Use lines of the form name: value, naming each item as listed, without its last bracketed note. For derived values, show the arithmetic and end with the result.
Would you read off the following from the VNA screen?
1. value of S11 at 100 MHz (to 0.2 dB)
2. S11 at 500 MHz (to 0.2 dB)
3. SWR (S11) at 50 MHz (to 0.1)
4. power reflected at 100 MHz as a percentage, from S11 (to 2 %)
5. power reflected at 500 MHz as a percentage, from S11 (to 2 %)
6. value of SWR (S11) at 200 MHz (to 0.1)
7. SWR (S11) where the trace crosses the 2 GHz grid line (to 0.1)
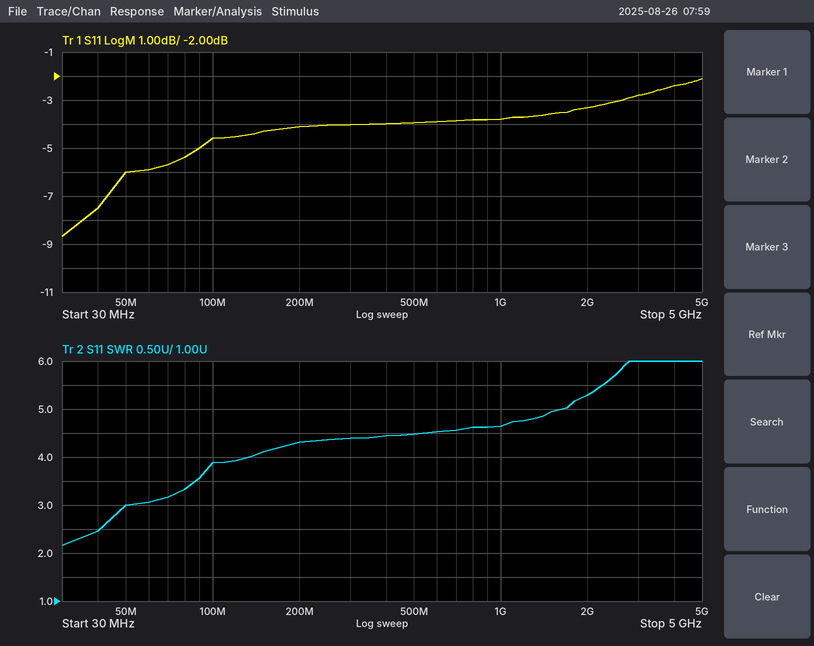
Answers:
value of S11 at 100 MHz: -4.6 dB
S11 at 500 MHz: -4.0 dB
SWR (S11) at 50 MHz: 3.0
power reflected at 100 MHz as a percentage, from S11: 10^(-4.6/10) ≈ 34.7 %, so 34 % to the nearest 2 %
power reflected at 500 MHz as a percentage, from S11: 10^(-4/10) ≈ 40 %
value of SWR (S11) at 200 MHz: 4.3
SWR (S11) where the trace crosses the 2 GHz grid line: 5.3
